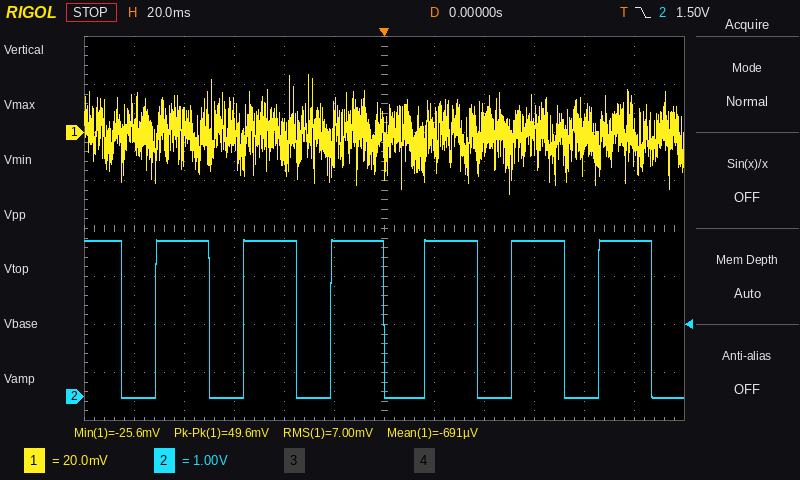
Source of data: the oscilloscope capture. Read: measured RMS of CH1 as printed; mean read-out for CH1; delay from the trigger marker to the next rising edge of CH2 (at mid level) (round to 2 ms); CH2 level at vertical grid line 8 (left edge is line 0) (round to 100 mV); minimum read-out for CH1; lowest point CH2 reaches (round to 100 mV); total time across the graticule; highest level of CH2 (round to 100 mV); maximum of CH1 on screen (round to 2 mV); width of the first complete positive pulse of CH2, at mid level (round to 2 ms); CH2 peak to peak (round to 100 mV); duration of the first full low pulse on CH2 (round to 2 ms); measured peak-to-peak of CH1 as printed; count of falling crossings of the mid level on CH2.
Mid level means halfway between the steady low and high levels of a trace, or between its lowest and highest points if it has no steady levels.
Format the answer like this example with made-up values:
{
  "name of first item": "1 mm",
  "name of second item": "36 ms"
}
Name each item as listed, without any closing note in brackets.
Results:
{
  "measured RMS of CH1 as printed": "7.00 mV",
  "mean read-out for CH1": "-691 µV",
  "delay from the trigger marker to the next rising edge of CH2 (at mid level)": "16 ms",
  "CH2 level at vertical grid line 8 (left edge is line 0)": "0.0 V",
  "minimum read-out for CH1": "-25.6 mV",
  "lowest point CH2 reaches": "0.0 V",
  "total time across the graticule": "240 ms",
  "highest level of CH2": "3.3 V",
  "maximum of CH1 on screen": "24 mV",
  "width of the first complete positive pulse of CH2, at mid level": "22 ms",
  "CH2 peak to peak": "3.3 V",
  "duration of the first full low pulse on CH2": "14 ms",
  "measured peak-to-peak of CH1 as printed": "49.6 mV",
  "count of falling crossings of the mid level on CH2": "7"
}
